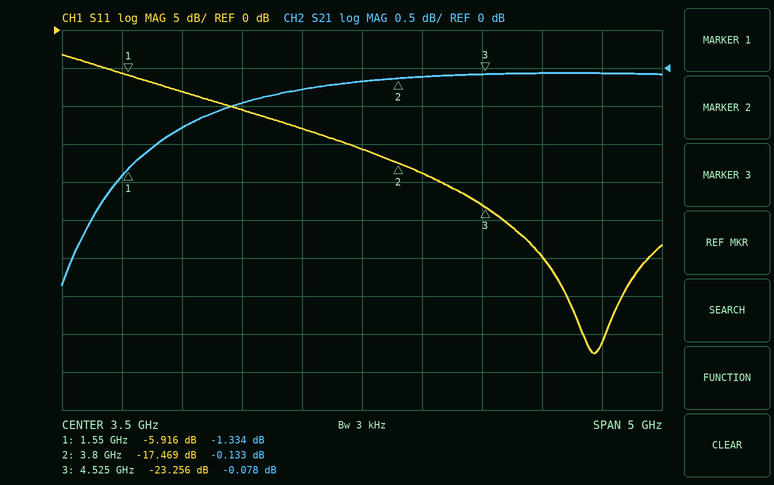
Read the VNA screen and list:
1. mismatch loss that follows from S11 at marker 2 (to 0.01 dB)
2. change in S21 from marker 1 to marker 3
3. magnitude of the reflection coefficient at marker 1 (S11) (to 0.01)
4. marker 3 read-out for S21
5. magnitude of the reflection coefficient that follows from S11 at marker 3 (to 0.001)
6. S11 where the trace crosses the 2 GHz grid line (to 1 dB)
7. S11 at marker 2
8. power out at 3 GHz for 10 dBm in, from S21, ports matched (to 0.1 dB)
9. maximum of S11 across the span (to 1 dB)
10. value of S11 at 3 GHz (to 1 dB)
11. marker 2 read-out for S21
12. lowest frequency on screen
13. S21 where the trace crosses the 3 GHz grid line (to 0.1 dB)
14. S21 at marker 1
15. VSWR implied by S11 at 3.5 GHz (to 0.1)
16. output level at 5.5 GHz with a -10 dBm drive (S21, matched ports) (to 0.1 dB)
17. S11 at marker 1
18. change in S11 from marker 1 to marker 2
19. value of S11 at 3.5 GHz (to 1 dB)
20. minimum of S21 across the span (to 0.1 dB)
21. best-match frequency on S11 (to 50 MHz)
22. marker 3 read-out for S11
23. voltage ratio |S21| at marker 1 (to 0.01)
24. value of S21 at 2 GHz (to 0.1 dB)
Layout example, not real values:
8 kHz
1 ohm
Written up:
0.08 dB
1.256 dB
0.51
-0.078 dB
0.069
-8 dB
-17.469 dB
9.7 dBm
-3 dB
-13 dB
-0.133 dB
1 GHz
-0.3 dB
-1.334 dB
1.4
-10.1 dBm
-5.916 dB
-11.553 dB
-16 dB
-2.9 dB
5.45 GHz
-23.256 dB
0.86
-0.8 dB
